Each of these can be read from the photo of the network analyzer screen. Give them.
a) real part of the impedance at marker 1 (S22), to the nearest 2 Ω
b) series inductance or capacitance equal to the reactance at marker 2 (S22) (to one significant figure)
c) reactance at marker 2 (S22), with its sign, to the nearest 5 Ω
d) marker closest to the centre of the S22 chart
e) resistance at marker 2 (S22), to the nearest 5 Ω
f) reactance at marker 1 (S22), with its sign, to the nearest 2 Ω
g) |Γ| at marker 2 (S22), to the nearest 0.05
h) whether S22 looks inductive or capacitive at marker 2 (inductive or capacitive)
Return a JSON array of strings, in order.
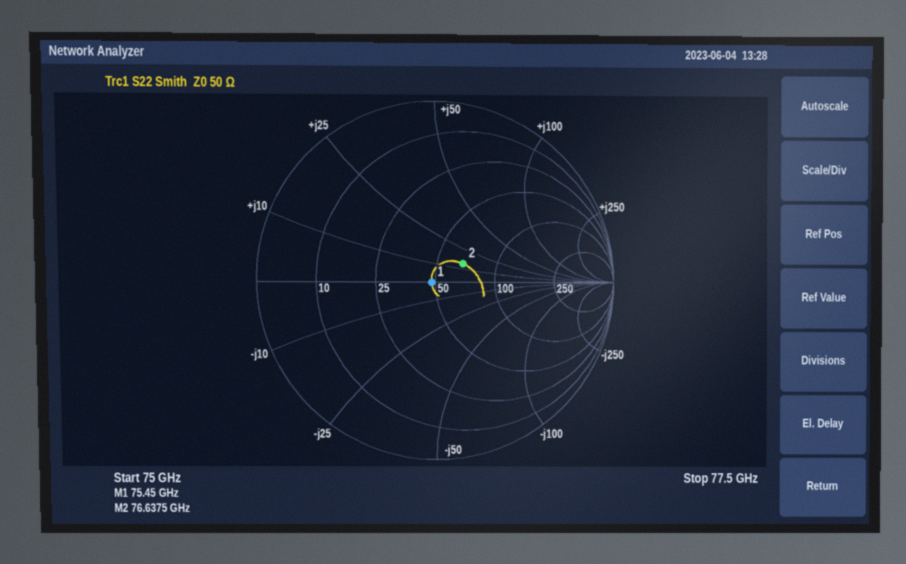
["48 Ω", "30 pH", "+15 Ω", "marker 1", "65 Ω", "0 Ω", "0.20", "inductive"]
